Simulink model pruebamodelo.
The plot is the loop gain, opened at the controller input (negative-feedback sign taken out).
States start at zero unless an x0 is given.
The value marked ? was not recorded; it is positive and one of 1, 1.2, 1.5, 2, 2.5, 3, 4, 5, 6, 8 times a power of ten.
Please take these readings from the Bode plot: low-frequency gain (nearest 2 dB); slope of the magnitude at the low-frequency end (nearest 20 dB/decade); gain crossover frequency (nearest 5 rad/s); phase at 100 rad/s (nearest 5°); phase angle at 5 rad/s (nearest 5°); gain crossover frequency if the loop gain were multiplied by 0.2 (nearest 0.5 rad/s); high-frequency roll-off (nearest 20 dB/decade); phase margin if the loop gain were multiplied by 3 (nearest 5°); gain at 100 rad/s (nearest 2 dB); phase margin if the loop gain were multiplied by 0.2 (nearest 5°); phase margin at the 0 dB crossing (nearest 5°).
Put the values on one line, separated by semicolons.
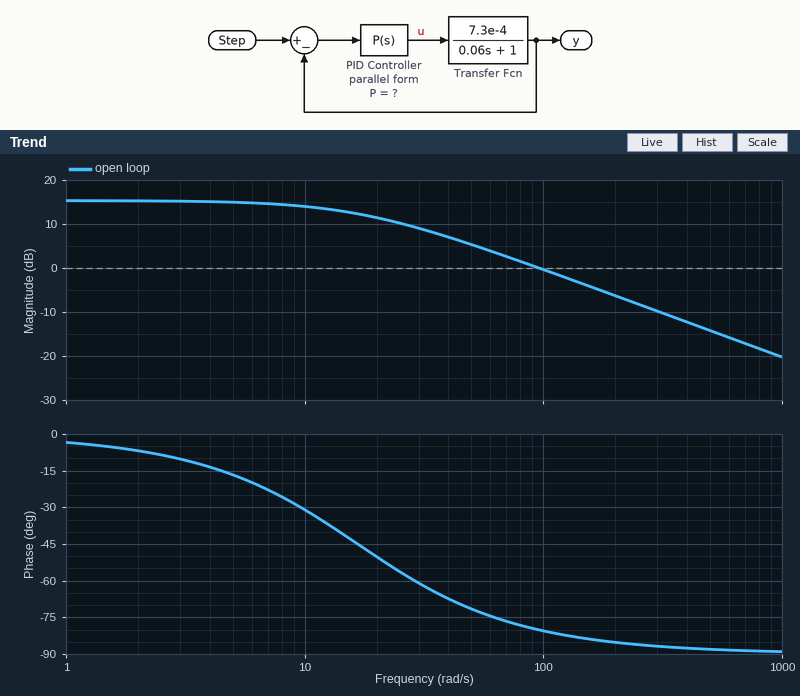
16 dB; 0 dB/decade; 95 rad/s; -80°; -15°; 10.0 rad/s; -20 dB/decade; 95°; 0 dB; 150°; 100°
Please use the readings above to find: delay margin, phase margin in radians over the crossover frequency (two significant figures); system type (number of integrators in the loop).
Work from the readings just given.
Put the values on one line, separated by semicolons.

0.018 s; 0
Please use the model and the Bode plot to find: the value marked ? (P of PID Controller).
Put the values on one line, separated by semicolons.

8000
